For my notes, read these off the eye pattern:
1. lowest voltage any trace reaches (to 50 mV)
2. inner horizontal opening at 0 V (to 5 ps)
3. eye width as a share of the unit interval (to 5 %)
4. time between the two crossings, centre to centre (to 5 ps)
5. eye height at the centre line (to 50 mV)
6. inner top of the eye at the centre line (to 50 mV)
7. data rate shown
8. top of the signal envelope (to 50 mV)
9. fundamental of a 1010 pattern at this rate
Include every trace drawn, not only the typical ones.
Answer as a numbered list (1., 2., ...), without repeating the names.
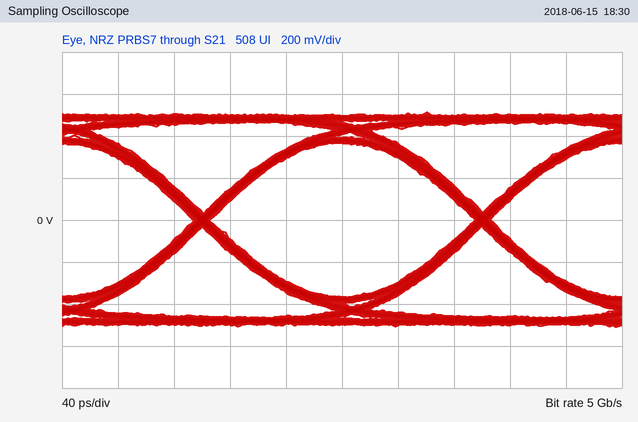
1. -500 mV
2. 190 ps
3. 95 %
4. 200 ps
5. 750 mV
6. 350 mV
7. 5 Gb/s
8. 500 mV
9. 2.5 GHz
